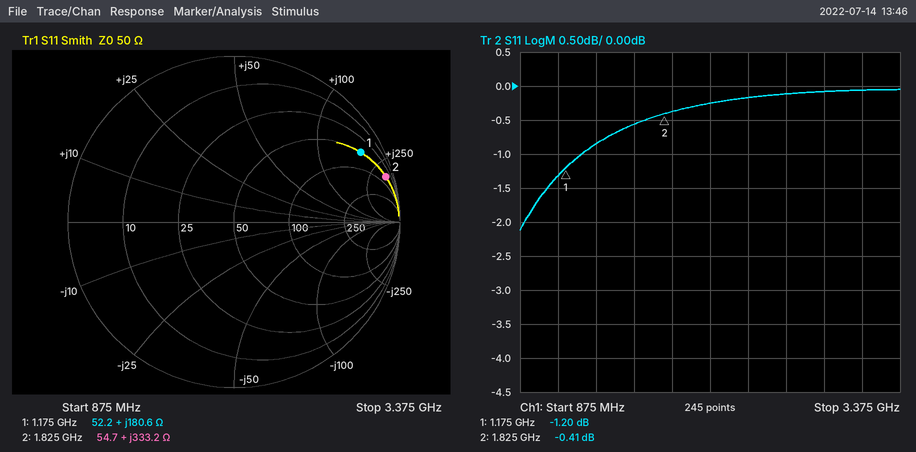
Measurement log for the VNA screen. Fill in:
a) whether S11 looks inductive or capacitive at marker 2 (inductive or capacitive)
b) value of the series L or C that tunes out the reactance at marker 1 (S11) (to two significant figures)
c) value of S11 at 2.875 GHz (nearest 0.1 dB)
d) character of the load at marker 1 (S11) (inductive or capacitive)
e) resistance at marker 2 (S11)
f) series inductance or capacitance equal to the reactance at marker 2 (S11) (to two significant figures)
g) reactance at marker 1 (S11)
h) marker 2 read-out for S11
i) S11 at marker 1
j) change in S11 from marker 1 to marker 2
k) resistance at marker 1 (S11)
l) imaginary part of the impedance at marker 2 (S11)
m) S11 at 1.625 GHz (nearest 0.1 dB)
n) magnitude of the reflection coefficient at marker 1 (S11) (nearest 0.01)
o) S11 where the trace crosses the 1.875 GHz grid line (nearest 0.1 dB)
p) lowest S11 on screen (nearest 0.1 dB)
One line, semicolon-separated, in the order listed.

inductive; 750 fF; -0.1 dB; inductive; 54.7 Ω; 29 nH; +180.6 Ω; -0.41 dB; -1.20 dB; 0.79 dB; 52.2 Ω; +333.2 Ω; -0.6 dB; 0.87; -0.4 dB; -2.1 dB
